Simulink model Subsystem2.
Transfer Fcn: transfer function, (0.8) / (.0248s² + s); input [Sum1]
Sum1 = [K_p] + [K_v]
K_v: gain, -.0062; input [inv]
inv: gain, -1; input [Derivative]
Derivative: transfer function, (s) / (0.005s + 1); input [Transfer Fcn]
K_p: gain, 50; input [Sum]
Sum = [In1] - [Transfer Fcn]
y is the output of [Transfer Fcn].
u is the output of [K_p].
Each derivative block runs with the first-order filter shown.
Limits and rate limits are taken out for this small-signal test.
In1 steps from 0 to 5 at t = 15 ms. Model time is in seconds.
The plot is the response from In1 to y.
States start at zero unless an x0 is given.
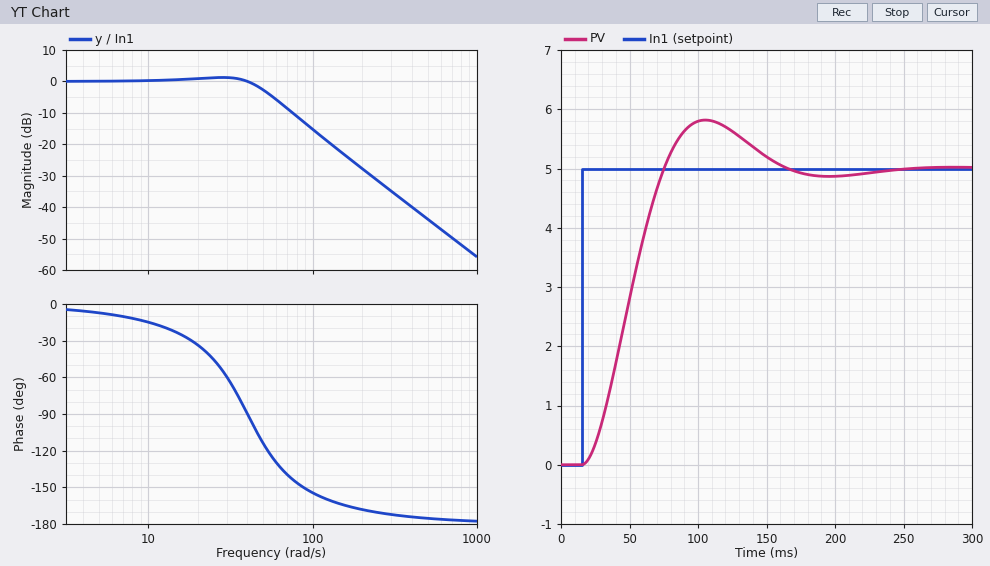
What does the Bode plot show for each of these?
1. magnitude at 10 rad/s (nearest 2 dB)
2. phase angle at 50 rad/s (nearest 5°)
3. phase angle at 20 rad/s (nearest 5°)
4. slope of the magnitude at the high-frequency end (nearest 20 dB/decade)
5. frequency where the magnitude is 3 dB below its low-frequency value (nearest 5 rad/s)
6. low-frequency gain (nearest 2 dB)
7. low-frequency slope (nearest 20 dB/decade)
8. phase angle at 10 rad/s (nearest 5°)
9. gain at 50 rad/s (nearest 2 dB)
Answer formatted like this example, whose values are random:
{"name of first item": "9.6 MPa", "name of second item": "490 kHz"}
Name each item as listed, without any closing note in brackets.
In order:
{"magnitude at 10 rad/s": "0 dB", "phase angle at 50 rad/s": "-115°", "phase angle at 20 rad/s": "-35°", "slope of the magnitude at the high-frequency end": "-40 dB/decade", "frequency where the magnitude is 3 dB below its low-frequency value": "50 rad/s", "low-frequency gain": "0 dB", "low-frequency slope": "0 dB/decade", "phase angle at 10 rad/s": "-15°", "gain at 50 rad/s": "-2 dB"}
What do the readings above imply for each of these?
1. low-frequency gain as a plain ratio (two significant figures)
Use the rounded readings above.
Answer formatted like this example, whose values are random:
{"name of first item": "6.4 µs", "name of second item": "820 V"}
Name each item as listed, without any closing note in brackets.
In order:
{"low-frequency gain as a plain ratio": "1.0"}
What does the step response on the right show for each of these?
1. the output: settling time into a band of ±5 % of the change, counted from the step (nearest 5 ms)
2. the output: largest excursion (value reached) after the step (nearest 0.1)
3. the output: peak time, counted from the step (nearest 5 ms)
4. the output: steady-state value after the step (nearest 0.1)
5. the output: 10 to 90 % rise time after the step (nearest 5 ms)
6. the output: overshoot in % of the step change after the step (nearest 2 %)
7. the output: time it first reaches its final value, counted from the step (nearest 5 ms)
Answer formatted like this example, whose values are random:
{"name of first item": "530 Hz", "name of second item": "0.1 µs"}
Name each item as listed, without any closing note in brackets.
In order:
{"the output: settling time into a band of ±5 % of the change, counted from the step": "130 ms", "the output: largest excursion (value reached) after the step": "5.8", "the output: peak time, counted from the step": "90 ms", "the output: steady-state value after the step": "5.0", "the output: 10 to 90 % rise time after the step": "40 ms", "the output: overshoot in % of the step change after the step": "16 %", "the output: time it first reaches its final value, counted from the step": "60 ms"}
